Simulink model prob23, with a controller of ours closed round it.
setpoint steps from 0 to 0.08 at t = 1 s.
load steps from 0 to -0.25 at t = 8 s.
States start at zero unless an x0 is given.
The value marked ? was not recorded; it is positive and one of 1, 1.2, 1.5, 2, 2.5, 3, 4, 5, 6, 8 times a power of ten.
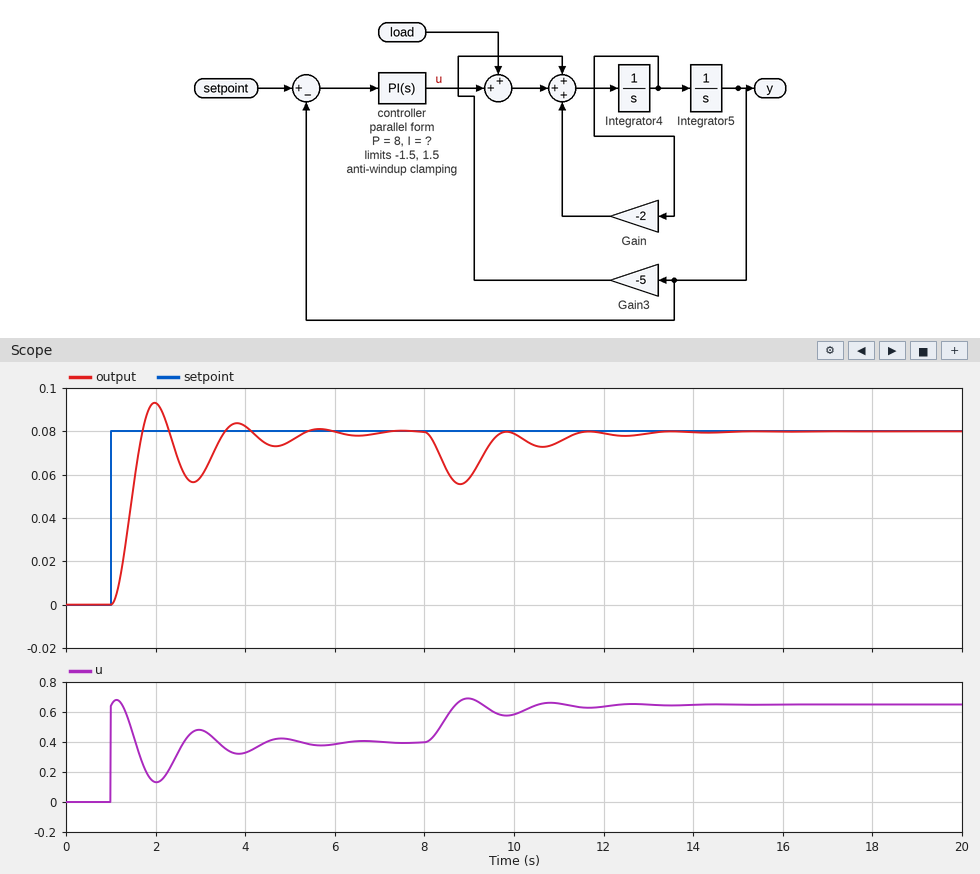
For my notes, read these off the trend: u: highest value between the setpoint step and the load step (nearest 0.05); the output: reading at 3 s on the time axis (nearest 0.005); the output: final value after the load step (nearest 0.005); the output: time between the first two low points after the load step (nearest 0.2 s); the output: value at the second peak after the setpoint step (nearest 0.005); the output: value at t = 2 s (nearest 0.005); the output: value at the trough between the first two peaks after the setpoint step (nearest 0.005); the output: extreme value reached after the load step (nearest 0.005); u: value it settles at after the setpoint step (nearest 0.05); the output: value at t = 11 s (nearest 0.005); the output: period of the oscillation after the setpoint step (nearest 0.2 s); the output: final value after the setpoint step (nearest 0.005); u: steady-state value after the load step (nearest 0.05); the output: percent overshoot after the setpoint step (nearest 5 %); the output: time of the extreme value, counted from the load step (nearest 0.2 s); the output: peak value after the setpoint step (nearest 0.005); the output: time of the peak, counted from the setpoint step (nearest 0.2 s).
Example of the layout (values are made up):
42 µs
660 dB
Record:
0.70
0.060
0.080
1.8 s
0.085
0.095
0.055
0.055
0.40
0.075
1.8 s
0.080
0.65
15 %
0.8 s
0.095
1.0 s
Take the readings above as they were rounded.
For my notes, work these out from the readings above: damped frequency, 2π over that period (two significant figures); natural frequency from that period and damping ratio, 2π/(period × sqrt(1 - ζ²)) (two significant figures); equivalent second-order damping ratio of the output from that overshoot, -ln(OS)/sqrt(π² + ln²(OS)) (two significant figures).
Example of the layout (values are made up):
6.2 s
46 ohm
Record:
3.5 rad/s
4.1 rad/s
0.52
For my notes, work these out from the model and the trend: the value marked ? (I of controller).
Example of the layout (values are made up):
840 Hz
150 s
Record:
8
